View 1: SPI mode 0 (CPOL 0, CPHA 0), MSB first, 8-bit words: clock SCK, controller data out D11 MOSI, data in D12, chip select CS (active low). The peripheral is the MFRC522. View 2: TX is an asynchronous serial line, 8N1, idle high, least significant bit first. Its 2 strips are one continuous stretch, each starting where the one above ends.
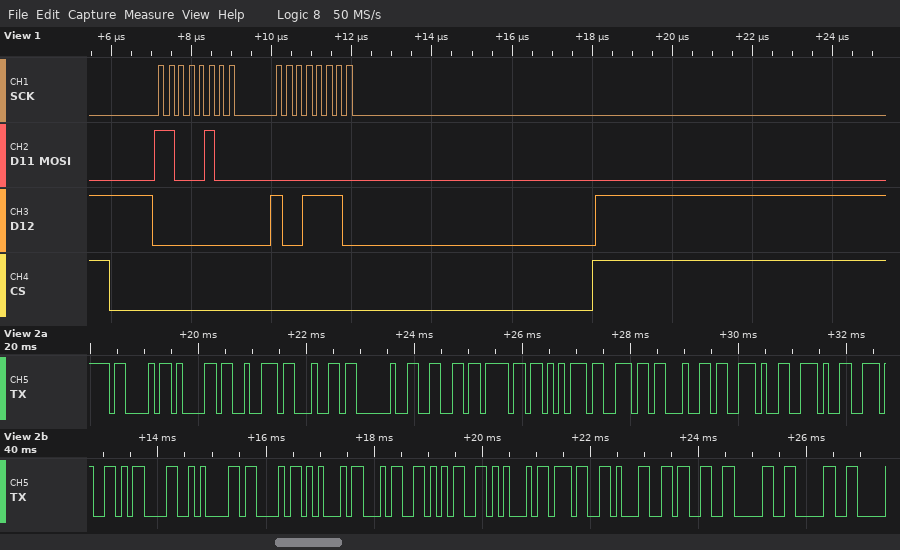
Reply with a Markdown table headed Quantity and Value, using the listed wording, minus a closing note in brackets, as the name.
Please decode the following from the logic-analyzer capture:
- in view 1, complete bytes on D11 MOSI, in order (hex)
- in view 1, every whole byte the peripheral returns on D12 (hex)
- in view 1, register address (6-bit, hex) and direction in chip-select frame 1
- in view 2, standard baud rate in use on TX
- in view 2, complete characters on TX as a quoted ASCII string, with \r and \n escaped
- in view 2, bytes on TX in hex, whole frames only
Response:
| Quantity | Value |
|---|---|
| in view 1, complete bytes on D11 MOSI, in order | C4 00 |
| in view 1, every whole byte the peripheral returns on D12 | 00 9E |
| in view 1, register address (6-bit, hex) and direction in chip-select frame 1 | 0x22 read |
| in view 2, standard baud rate in use on TX | 9600 baud |
| in view 2, complete characters on TX as a quoted ASCII string, with \r and \n escaped | "Card found...\r\nCE45E71300" |
| in view 2, bytes on TX in hex, whole frames only | 43 61 72 64 20 66 6F 75 6E 64 2E 2E 2E 0D 0A 43 45 34 35 45 37 31 33 30 30 |
